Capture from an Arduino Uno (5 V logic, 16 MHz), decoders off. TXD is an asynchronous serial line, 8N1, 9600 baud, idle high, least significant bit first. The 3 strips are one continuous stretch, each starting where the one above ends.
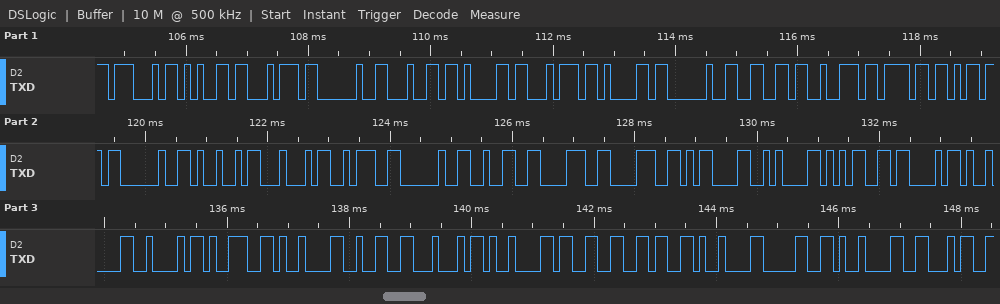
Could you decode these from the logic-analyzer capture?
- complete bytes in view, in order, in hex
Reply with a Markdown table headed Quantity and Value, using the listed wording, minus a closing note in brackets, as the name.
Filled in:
| Quantity | Value |
|---|---|
| complete bytes in view, in order, in hex | 47 65 74 20 64 61 74 61 20 66 72 6F 6D 20 49 44 3A 20 32 38 38 0D 0A 35 43 09 42 39 09 32 44 09 33 36 09 30 09 46 |
